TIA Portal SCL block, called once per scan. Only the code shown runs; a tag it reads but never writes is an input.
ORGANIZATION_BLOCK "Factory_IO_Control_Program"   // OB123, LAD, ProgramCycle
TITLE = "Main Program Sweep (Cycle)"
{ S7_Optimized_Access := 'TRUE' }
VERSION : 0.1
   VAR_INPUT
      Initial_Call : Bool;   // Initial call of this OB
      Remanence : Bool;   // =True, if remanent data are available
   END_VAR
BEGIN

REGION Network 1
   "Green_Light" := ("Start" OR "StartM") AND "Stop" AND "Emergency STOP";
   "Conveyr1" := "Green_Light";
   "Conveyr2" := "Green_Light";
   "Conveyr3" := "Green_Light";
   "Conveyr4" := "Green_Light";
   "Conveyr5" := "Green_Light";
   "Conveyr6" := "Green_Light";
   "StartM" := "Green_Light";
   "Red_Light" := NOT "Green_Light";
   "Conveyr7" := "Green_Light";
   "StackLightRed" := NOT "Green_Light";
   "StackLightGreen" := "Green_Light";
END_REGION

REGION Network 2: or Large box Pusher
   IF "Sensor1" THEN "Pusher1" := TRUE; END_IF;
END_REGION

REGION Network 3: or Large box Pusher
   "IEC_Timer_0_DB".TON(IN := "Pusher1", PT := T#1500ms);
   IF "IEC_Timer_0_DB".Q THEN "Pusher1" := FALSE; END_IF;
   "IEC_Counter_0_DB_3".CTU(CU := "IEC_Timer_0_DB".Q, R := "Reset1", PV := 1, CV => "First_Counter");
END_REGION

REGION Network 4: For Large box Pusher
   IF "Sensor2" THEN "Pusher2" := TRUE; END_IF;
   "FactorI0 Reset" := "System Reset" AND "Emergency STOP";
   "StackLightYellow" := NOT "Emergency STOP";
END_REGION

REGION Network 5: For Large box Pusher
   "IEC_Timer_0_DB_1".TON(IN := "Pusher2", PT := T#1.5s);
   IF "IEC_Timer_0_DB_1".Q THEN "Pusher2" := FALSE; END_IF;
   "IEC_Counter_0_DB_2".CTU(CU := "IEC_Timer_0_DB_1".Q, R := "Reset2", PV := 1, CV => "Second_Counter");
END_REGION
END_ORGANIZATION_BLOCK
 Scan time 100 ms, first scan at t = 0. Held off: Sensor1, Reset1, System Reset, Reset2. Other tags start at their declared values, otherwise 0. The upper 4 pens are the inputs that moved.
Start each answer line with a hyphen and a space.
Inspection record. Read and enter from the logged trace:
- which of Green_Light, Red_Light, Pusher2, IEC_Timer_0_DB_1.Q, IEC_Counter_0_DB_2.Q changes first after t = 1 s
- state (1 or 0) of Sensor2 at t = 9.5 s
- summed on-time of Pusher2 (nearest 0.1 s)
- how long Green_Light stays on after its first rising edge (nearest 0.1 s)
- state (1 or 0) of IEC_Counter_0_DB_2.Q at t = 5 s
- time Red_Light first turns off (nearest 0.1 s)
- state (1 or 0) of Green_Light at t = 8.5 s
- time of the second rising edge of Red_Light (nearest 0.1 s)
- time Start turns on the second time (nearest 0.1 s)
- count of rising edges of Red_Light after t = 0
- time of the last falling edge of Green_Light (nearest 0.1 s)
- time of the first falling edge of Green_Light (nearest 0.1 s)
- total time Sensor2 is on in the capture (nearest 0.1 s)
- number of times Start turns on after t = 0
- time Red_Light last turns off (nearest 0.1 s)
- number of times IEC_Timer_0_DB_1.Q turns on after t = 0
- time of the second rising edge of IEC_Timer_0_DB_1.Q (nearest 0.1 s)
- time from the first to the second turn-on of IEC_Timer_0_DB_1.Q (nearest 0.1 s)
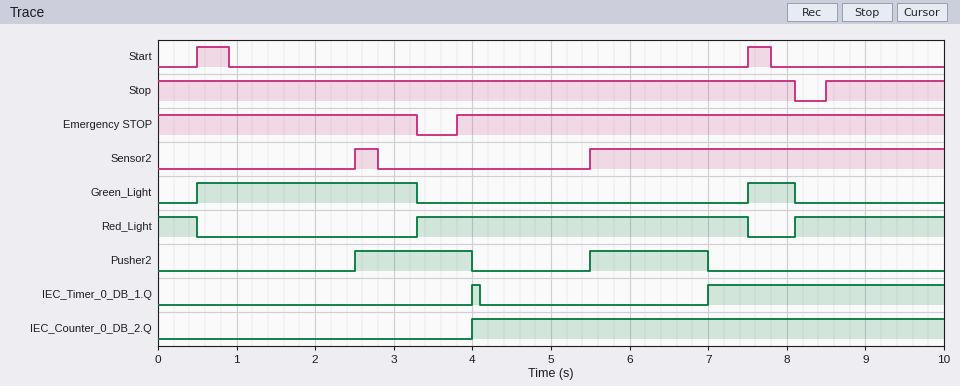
- Pusher2
- 1
- 3.0 s
- 2.8 s
- 1
- 0.5 s
- 0
- 8.1 s
- 7.5 s
- 2
- 8.1 s
- 3.3 s
- 4.8 s
- 2
- 7.5 s
- 2
- 7.0 s
- 3.0 s
